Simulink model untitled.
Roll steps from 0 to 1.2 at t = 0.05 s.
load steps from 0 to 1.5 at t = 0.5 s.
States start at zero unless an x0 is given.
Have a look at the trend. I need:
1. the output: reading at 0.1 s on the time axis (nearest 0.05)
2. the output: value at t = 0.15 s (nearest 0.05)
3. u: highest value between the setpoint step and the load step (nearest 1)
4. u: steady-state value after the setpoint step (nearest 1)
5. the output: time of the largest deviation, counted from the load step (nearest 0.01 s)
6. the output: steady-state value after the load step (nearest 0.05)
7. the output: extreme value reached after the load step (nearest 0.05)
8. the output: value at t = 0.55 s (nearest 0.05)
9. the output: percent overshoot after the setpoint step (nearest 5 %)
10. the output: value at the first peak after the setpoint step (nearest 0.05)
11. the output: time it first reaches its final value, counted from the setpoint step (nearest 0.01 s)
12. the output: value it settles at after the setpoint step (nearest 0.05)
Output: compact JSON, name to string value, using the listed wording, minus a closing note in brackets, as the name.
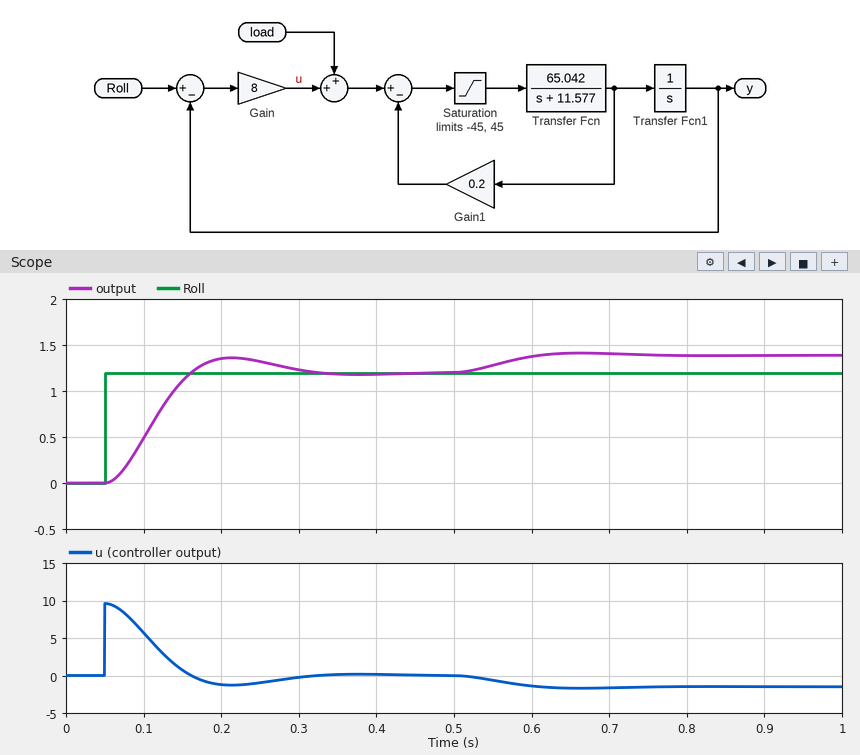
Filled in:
{"the output: reading at 0.1 s on the time axis": "0.50", "the output: value at t = 0.15 s": "1.10", "u: highest value between the setpoint step and the load step": "10", "u: steady-state value after the setpoint step": "0", "the output: time of the largest deviation, counted from the load step": "0.16 s", "the output: steady-state value after the load step": "1.40", "the output: extreme value reached after the load step": "1.40", "the output: value at t = 0.55 s": "1.30", "the output: percent overshoot after the setpoint step": "15 %", "the output: value at the first peak after the setpoint step": "1.35", "the output: time it first reaches its final value, counted from the setpoint step": "0.11 s", "the output: value it settles at after the setpoint step": "1.20"}
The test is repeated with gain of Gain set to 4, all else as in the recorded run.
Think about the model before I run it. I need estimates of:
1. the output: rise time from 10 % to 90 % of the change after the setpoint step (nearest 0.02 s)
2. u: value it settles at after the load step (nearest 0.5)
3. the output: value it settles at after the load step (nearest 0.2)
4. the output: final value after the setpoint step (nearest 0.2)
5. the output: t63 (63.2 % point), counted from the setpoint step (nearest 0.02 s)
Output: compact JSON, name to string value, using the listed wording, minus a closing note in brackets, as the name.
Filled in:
{"the output: rise time from 10 % to 90 % of the change after the setpoint step": "0.14 s", "u: value it settles at after the load step": "-1.5", "the output: value it settles at after the load step": "1.6", "the output: final value after the setpoint step": "1.2", "the output: t63 (63.2 % point), counted from the setpoint step": "0.12 s"}
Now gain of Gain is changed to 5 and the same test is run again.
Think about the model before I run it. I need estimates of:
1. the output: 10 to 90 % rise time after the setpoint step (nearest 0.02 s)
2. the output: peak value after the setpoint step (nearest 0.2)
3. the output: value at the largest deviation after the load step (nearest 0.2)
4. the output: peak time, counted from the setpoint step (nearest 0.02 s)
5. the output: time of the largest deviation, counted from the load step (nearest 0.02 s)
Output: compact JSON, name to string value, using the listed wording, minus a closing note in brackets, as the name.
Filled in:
{"the output: 10 to 90 % rise time after the setpoint step": "0.12 s", "the output: peak value after the setpoint step": "1.2", "the output: value at the largest deviation after the load step": "1.6", "the output: peak time, counted from the setpoint step": "0.24 s", "the output: time of the largest deviation, counted from the load step": "0.24 s"}
